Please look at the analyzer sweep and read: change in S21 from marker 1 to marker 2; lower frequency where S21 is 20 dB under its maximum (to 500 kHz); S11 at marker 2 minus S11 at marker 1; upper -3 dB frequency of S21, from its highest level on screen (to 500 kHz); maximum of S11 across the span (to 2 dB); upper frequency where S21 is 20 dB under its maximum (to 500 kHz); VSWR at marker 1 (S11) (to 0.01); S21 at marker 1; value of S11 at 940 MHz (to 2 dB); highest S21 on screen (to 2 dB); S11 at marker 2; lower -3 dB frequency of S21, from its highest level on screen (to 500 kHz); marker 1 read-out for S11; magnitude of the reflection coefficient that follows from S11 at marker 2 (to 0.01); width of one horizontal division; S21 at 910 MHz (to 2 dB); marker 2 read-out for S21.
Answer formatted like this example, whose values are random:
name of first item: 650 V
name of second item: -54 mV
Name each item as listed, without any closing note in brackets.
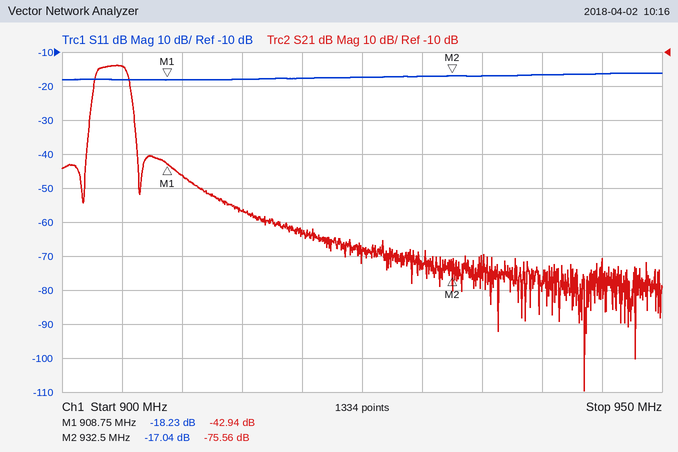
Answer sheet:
change in S21 from marker 1 to marker 2: -32.62 dB
lower frequency where S21 is 20 dB under its maximum: 902.0 MHz
S11 at marker 2 minus S11 at marker 1: 1.19 dB
upper -3 dB frequency of S21, from its highest level on screen: 905.5 MHz
maximum of S11 across the span: -16 dB
upper frequency where S21 is 20 dB under its maximum: 906.0 MHz
VSWR at marker 1 (S11): 1.28
S21 at marker 1: -42.94 dB
value of S11 at 940 MHz: -16 dB
highest S21 on screen: -14 dB
S11 at marker 2: -17.04 dB
lower -3 dB frequency of S21, from its highest level on screen: 903.0 MHz
marker 1 read-out for S11: -18.23 dB
magnitude of the reflection coefficient that follows from S11 at marker 2: 0.14
width of one horizontal division: 5 MHz
S21 at 910 MHz: -46 dB
marker 2 read-out for S21: -75.56 dB
